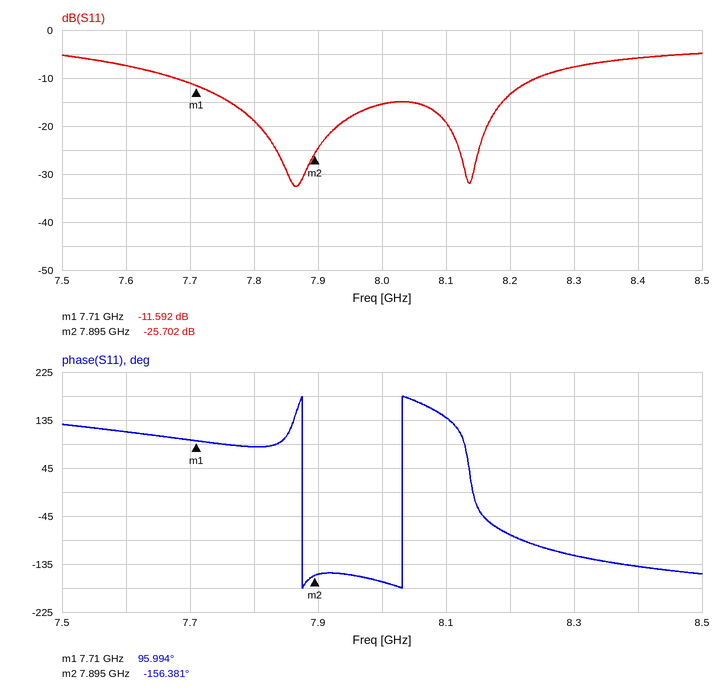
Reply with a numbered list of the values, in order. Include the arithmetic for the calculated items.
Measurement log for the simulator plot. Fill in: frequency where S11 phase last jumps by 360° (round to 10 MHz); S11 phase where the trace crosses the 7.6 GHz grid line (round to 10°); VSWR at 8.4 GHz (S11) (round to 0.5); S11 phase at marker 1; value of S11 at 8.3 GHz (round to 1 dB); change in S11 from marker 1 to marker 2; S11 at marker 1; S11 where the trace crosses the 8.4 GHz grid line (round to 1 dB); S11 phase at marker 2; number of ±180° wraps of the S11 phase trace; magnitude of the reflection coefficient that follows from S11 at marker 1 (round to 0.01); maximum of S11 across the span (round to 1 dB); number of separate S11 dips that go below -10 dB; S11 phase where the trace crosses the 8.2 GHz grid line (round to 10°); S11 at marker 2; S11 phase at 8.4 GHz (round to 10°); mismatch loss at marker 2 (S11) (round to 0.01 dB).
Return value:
1. 8.03 GHz
2. 110°
3. |Γ| = 10^(-6/20) = 0.5012; VSWR = (1 + 0.5012)/(1 − 0.5012) ≈ 3.0
4. 95.994°
5. -8 dB
6. -25.702 − (-11.592) = -14.110 dB
7. -11.592 dB
8. -6 dB
9. -156.381°
10. 2
11. 10^(-11.592/20) ≈ 0.26
12. -5 dB
13. 2
14. -80°
15. -25.702 dB
16. -140°
17. −10 log10(1 − 10^(-25.702/10)) ≈ 0.01 dB
